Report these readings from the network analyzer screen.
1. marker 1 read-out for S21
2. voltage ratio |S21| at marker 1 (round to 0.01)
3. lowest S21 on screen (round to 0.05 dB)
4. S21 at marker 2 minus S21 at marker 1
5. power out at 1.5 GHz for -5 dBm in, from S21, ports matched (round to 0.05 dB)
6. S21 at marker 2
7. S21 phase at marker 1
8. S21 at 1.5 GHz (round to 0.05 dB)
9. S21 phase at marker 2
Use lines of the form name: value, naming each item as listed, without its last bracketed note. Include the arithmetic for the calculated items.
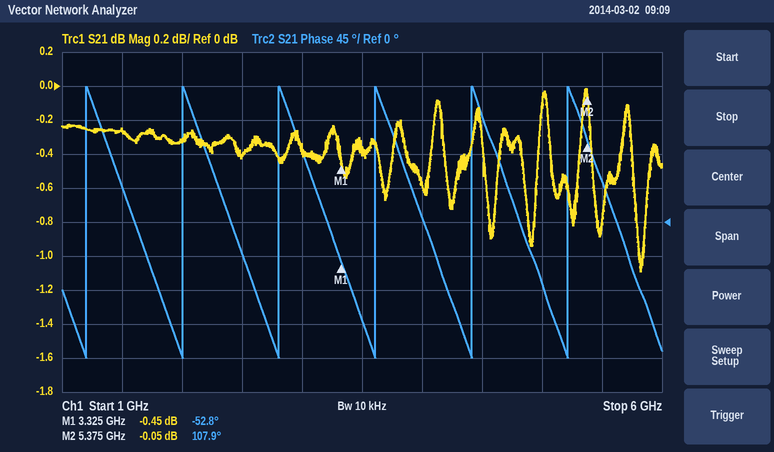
marker 1 read-out for S21: -0.45 dB
voltage ratio |S21| at marker 1: 10^(-0.45/20) ≈ 0.95
lowest S21 on screen: -1.10 dB
S21 at marker 2 minus S21 at marker 1: -0.05 − (-0.45) = 0.40 dB
power out at 1.5 GHz for -5 dBm in, from S21, ports matched: -5 dBm + (-0.25 dB) = -5.25 dBm
S21 at marker 2: -0.05 dB
S21 phase at marker 1: -52.8°
S21 at 1.5 GHz: -0.25 dB
S21 phase at marker 2: 107.9°
